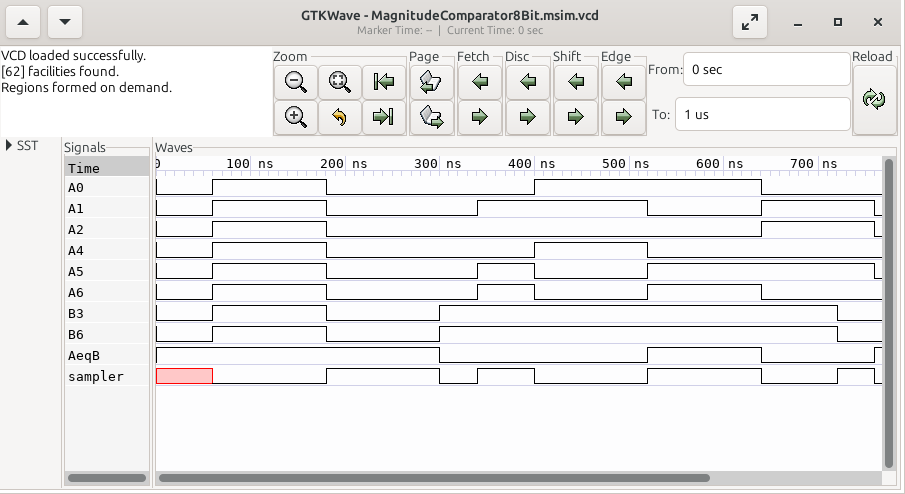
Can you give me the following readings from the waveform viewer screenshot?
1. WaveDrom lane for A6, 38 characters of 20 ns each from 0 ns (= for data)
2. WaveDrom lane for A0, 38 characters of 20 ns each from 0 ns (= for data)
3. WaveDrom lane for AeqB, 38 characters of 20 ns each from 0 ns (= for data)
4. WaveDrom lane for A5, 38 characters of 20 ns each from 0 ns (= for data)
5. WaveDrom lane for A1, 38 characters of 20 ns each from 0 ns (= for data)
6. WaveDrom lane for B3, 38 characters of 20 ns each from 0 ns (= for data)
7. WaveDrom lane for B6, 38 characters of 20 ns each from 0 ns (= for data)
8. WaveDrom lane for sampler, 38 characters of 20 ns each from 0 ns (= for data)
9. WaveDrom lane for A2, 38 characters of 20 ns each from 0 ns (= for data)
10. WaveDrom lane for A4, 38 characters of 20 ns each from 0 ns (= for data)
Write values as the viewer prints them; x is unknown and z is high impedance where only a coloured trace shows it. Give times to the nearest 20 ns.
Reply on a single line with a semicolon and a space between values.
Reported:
{name: 'A6', wave: '0..1.....0.......1..0.....1.....0.....'}; {name: 'A0', wave: '0..1.....0..........1...........0.....'}; {name: 'AeqB', wave: '1..............0..........1.....0.....'}; {name: 'A5', wave: '0..1.....0.......1..0.....1...........'}; {name: 'A1', wave: '0..1.....0.......1........0.....1.....'}; {name: 'B3', wave: '0..1.....0.....1....................0.'}; {name: 'B6', wave: '0..1.....0.....1....................0.'}; {name: 'sampler', wave: 'x..0.....1.....0.1..0.....1.....0...1.'}; {name: 'A2', wave: '0..1.....0......................1.....'}; {name: 'A4', wave: '0..1.....0..........1.....0...........'}
